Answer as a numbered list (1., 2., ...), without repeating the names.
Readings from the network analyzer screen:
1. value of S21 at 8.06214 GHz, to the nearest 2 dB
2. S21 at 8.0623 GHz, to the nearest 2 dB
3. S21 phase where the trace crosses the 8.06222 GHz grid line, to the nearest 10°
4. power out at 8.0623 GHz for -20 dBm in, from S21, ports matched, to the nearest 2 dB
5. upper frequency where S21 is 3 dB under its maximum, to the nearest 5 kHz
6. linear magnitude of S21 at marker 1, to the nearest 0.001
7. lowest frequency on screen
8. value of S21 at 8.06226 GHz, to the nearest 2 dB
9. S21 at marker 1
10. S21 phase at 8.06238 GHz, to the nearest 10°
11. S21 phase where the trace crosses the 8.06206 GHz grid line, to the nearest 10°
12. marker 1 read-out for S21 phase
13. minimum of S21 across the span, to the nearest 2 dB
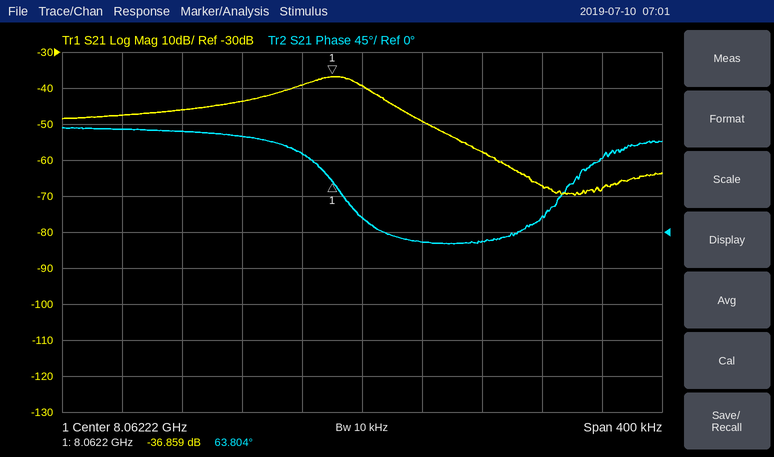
1. -44 dB
2. -58 dB
3. 20°
4. -78 dBm
5. 8.062220 GHz
6. 0.014
7. 8.06202 GHz
8. -50 dB
9. -36.859 dB
10. 90°
11. 130°
12. 63.804°
13. -70 dB
